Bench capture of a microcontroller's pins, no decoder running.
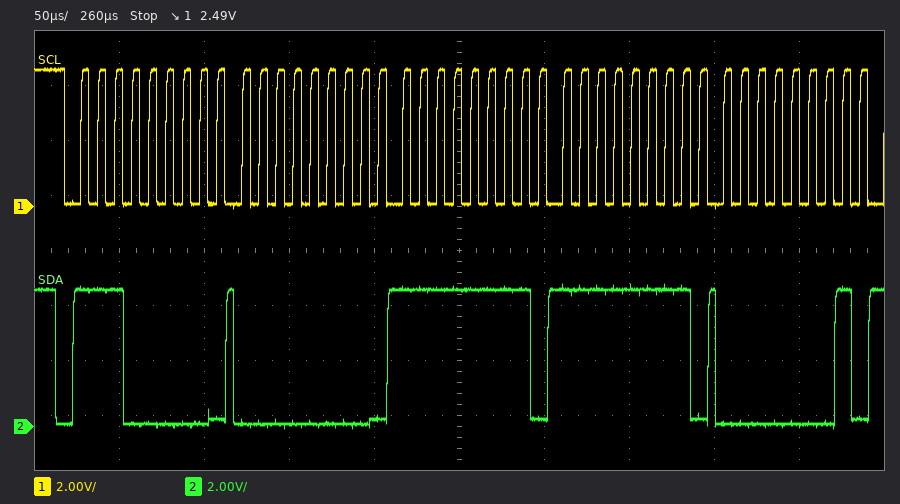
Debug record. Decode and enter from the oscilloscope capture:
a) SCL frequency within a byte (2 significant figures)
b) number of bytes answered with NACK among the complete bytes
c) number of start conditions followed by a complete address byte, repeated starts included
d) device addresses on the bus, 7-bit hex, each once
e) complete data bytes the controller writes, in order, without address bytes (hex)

100 kHz
0
1
0x70
00 FF FF 01
